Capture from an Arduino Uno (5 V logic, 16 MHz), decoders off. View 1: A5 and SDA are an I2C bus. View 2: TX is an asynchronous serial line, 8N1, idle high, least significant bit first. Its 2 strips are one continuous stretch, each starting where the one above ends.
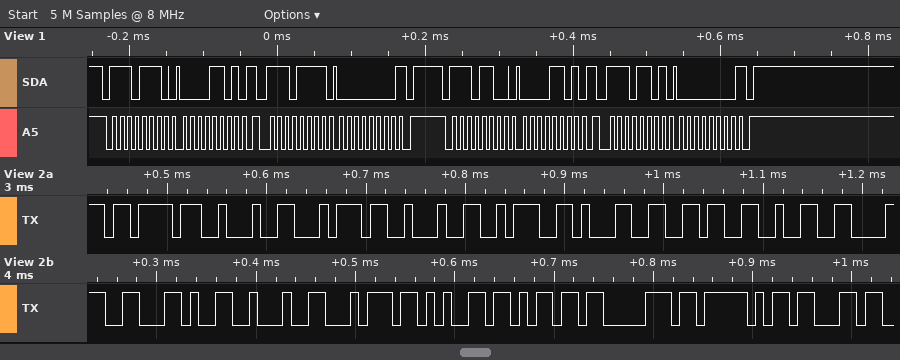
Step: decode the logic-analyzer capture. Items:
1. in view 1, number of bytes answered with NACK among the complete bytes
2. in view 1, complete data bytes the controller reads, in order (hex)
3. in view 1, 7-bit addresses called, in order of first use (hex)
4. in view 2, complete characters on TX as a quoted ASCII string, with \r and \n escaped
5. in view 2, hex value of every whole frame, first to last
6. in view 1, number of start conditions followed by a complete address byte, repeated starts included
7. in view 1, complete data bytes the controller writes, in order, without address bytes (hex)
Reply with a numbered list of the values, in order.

1. 2
2. 00 00
3. 0x77 0x76
4. "{\"t\":1628,\"temp_c"
5. 7B 22 74 22 3A 31 36 32 38 2C 22 74 65 6D 70 5F 63
6. 4
7. 0D 0D
